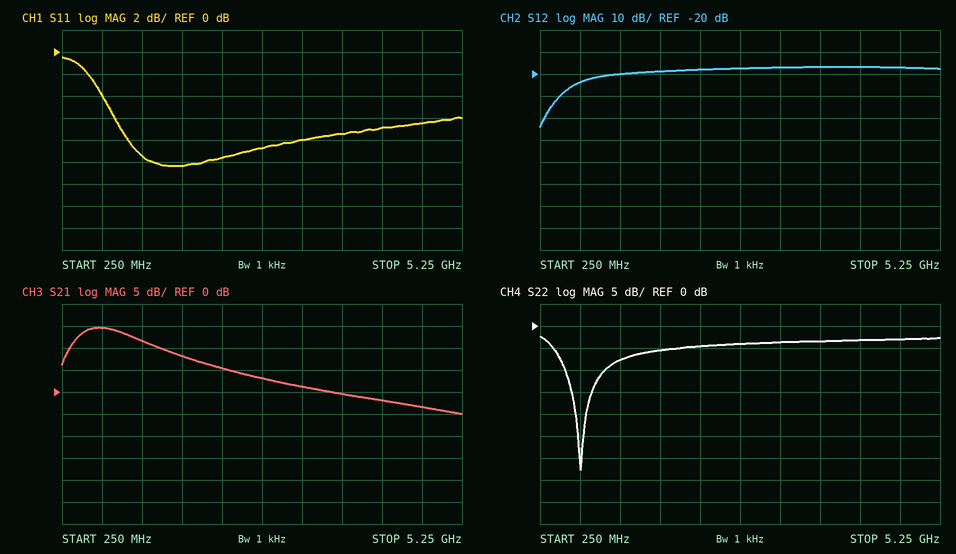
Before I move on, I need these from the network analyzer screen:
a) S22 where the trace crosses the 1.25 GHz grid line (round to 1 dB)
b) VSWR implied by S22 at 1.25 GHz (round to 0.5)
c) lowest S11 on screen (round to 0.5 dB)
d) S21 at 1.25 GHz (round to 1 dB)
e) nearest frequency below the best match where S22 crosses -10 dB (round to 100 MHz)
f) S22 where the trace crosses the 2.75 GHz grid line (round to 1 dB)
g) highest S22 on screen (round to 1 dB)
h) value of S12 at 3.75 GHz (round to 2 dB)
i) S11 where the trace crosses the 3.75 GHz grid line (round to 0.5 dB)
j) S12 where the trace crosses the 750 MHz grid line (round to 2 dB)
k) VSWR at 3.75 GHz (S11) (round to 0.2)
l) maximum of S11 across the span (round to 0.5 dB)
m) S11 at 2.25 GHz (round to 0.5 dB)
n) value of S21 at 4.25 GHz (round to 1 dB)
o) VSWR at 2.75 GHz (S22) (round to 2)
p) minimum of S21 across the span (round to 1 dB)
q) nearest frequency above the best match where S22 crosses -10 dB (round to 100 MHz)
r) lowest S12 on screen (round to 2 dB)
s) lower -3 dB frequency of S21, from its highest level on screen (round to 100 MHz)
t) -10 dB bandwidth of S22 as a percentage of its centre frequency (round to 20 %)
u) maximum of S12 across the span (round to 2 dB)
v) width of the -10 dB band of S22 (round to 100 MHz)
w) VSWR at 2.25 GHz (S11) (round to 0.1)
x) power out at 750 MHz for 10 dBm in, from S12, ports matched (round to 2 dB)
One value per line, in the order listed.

-8 dB
2.5
-10.5 dB
12 dB
600 MHz
-4 dB
-2 dB
-16 dB
-7.5 dB
-24 dB
2.4
-0.5 dB
-9.5 dB
-2 dB
4
-5 dB
1.1 GHz
-44 dB
400 MHz
60 %
-16 dB
500 MHz
2.0
-14 dBm
